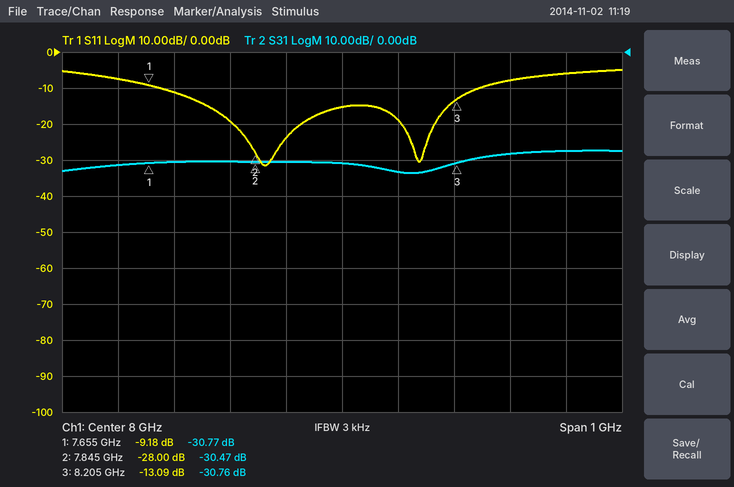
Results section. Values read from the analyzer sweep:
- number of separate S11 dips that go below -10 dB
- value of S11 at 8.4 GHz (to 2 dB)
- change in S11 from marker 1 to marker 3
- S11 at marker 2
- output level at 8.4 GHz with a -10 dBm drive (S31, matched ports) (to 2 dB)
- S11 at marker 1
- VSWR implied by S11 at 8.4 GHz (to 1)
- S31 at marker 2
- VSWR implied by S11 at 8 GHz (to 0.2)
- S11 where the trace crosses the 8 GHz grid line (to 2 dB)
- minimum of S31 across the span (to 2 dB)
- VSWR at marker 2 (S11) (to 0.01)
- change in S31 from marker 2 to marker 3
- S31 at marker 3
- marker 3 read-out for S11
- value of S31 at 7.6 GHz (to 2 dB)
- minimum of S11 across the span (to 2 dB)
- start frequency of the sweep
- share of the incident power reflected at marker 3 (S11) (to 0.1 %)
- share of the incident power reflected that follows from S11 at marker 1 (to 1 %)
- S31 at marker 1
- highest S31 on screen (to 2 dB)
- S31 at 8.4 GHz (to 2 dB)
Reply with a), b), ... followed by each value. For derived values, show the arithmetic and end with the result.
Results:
a) 2
b) -6 dB
c) -13.09 − (-9.18) = -3.91 dB
d) -28.00 dB
e) -10 dBm + (-28 dB) = -38 dBm
f) -9.18 dB
g) |Γ| = 10^(-6/20) = 0.5012; VSWR = (1 + 0.5012)/(1 − 0.5012) ≈ 3
h) -30.47 dB
i) |Γ| = 10^(-16/20) = 0.1585; VSWR = (1 + 0.1585)/(1 − 0.1585) ≈ 1.4
j) -16 dB
k) -34 dB
l) (1 + 0.0398)/(1 − 0.0398) ≈ 1.08
m) -30.76 − (-30.47) = -0.29 dB
n) -30.76 dB
o) -13.09 dB
p) -32 dB
q) -32 dB
r) 7.5 GHz
s) 10^(-13.09/10) ≈ 4.9 %
t) 10^(-9.18/10) ≈ 12 %
u) -30.77 dB
v) -28 dB
w) -28 dB
